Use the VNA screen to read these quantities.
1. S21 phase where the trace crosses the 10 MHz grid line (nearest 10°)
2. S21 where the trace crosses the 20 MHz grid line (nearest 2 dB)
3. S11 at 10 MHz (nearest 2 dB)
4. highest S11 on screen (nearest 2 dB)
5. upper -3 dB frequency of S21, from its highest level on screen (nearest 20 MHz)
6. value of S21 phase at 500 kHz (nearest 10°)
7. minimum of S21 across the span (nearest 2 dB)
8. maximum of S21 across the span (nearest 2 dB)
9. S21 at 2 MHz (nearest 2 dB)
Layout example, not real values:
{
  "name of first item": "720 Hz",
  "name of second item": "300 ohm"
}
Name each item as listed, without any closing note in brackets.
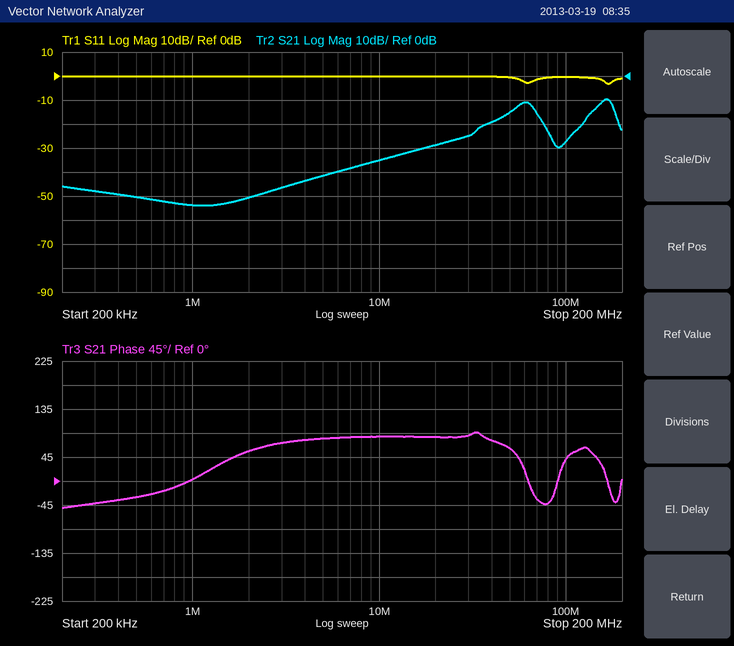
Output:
{
  "S21 phase where the trace crosses the 10 MHz grid line": "80°",
  "S21 where the trace crosses the 20 MHz grid line": "-28 dB",
  "S11 at 10 MHz": "0 dB",
  "highest S11 on screen": "0 dB",
  "upper -3 dB frequency of S21, from its highest level on screen": "180 MHz",
  "value of S21 phase at 500 kHz": "-30°",
  "minimum of S21 across the span": "-54 dB",
  "maximum of S21 across the span": "-10 dB",
  "S21 at 2 MHz": "-50 dB"
}
